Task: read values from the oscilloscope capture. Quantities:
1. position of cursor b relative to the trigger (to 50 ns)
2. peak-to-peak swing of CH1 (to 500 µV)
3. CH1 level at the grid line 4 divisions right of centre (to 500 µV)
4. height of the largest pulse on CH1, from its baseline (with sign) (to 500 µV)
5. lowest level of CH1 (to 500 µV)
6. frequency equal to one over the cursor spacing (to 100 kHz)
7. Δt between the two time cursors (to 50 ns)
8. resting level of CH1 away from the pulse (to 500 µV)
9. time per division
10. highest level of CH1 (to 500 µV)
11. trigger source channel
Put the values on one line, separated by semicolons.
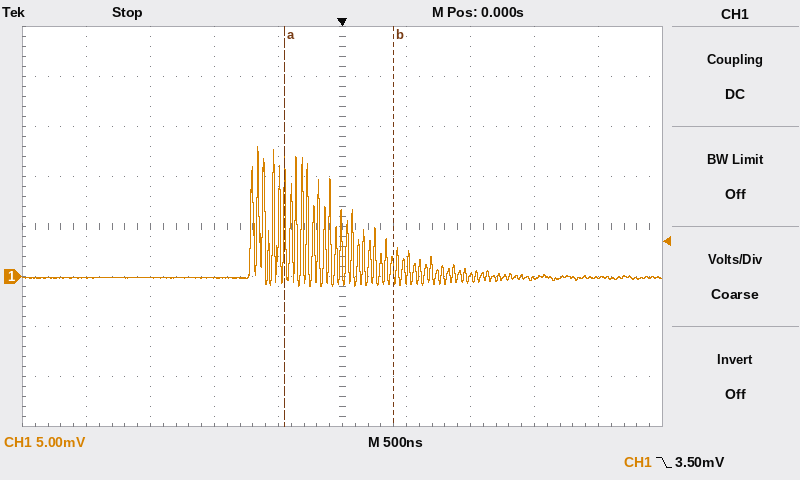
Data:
+400 ns; 14.0 mV; 0.0 mV; +13.0 mV; -1.0 mV; 1.2 MHz; 850 ns; 0.0 mV; 500 ns; 13.0 mV; CH1
